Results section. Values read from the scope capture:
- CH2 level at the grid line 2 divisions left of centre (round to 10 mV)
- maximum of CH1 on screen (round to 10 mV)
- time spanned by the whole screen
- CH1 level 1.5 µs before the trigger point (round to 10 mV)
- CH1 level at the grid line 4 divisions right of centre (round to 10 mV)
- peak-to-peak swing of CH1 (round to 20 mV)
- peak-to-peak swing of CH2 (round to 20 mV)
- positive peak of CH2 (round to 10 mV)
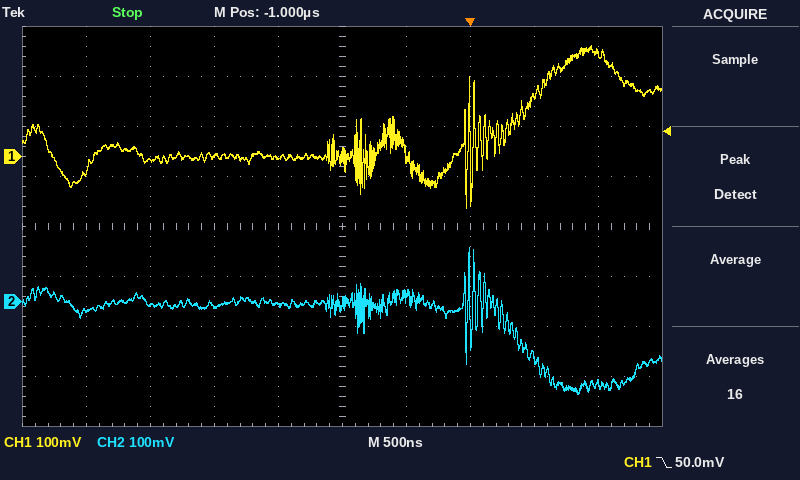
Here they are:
-10 mV
220 mV
5 µs
0 mV
210 mV
320 mV
300 mV
110 mV
